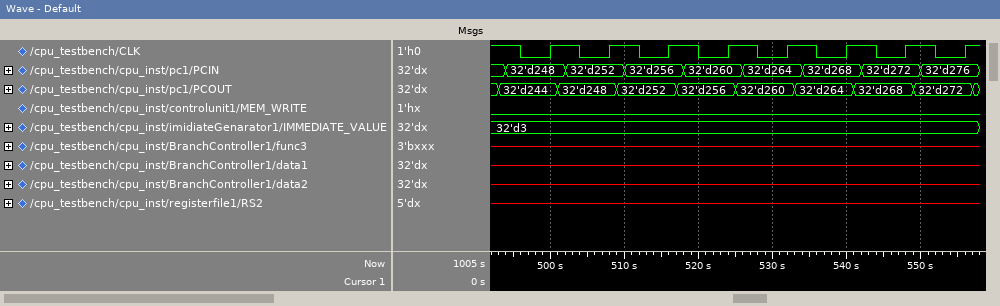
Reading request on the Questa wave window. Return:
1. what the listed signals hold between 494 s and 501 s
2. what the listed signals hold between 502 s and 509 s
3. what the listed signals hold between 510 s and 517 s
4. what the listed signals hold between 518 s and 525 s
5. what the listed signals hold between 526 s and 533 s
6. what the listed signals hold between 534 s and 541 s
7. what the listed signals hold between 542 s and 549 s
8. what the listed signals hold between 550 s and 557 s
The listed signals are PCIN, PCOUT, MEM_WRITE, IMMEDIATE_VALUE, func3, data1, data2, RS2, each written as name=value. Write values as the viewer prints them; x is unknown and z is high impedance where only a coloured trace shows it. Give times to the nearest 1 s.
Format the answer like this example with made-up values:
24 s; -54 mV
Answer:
PCIN=32'd248, PCOUT=32'd244, MEM_WRITE=0, IMMEDIATE_VALUE=32'd3, func3=x, data1=x, data2=x, RS2=x; PCIN=32'd252, PCOUT=32'd248, MEM_WRITE=0, IMMEDIATE_VALUE=32'd3, func3=x, data1=x, data2=x, RS2=x; PCIN=32'd256, PCOUT=32'd252, MEM_WRITE=0, IMMEDIATE_VALUE=32'd3, func3=x, data1=x, data2=x, RS2=x; PCIN=32'd260, PCOUT=32'd256, MEM_WRITE=0, IMMEDIATE_VALUE=32'd3, func3=x, data1=x, data2=x, RS2=x; PCIN=32'd264, PCOUT=32'd260, MEM_WRITE=0, IMMEDIATE_VALUE=32'd3, func3=x, data1=x, data2=x, RS2=x; PCIN=32'd268, PCOUT=32'd264, MEM_WRITE=0, IMMEDIATE_VALUE=32'd3, func3=x, data1=x, data2=x, RS2=x; PCIN=32'd272, PCOUT=32'd268, MEM_WRITE=0, IMMEDIATE_VALUE=32'd3, func3=x, data1=x, data2=x, RS2=x; PCIN=32'd276, PCOUT=32'd272, MEM_WRITE=0, IMMEDIATE_VALUE=32'd3, func3=x, data1=x, data2=x, RS2=x
